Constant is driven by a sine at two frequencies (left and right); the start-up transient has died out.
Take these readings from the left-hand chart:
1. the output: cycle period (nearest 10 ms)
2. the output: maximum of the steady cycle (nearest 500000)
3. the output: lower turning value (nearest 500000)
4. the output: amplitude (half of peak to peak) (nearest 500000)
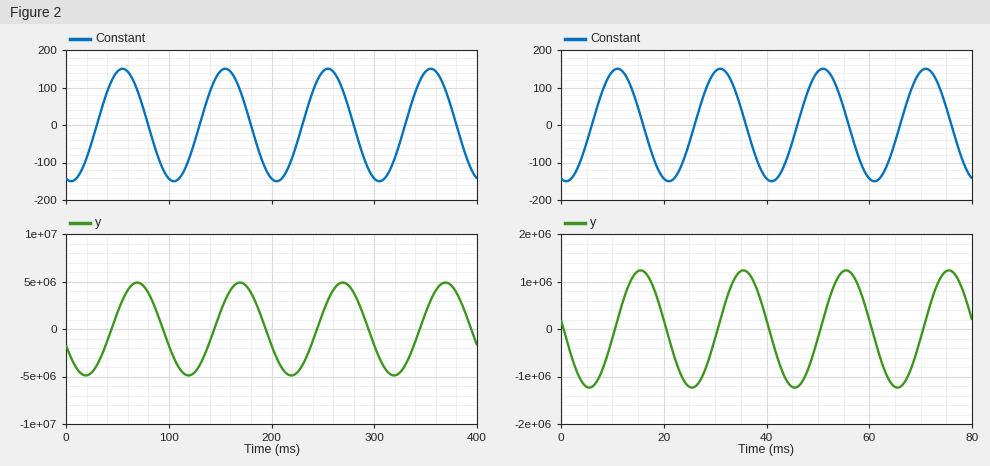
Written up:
100 ms
5000000
-5000000
5000000
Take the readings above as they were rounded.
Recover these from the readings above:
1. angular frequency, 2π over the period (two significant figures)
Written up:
0.063 rad/ms
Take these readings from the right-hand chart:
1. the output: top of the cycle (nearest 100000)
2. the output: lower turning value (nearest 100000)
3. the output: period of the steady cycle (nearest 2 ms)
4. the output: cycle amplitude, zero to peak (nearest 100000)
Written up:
1200000
-1200000
20 ms
1200000
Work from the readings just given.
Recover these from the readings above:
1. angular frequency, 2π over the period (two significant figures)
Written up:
0.31 rad/ms
